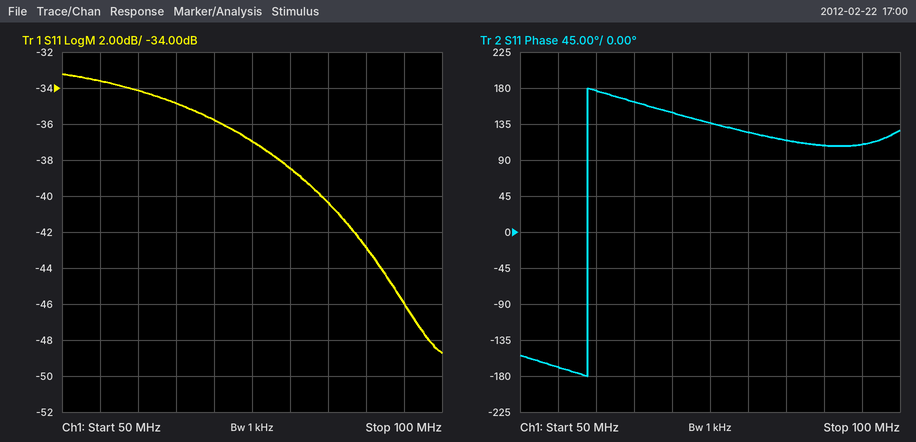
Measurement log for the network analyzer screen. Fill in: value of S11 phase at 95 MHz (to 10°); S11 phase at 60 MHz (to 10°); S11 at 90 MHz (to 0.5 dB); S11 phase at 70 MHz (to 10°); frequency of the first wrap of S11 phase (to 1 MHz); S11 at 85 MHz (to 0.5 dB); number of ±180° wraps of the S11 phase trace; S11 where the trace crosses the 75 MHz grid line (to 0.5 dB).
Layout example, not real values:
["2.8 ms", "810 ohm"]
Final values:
["110°", "180°", "-43.0 dB", "150°", "59 MHz", "-40.5 dB", "1", "-37.0 dB"]
